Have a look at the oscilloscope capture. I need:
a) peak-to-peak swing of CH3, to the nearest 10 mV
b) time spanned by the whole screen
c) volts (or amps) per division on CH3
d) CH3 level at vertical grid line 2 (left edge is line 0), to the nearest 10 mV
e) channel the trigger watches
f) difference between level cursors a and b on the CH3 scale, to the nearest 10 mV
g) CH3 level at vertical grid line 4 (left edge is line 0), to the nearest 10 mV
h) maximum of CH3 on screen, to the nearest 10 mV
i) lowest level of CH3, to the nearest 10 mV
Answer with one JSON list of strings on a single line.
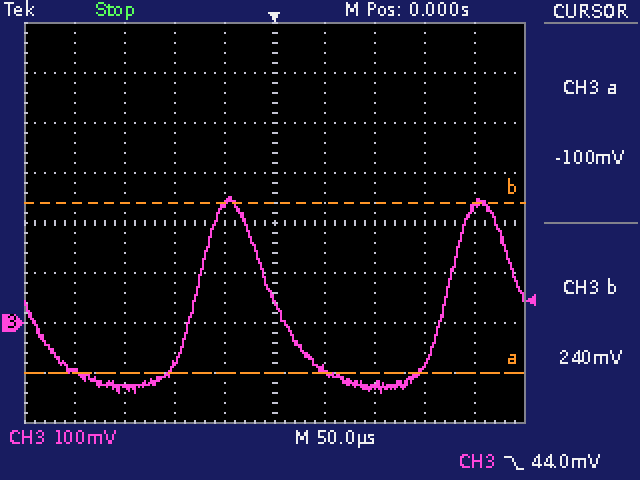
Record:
["390 mV", "500 µs", "100 mV", "-130 mV", "CH3", "340 mV", "240 mV", "250 mV", "-140 mV"]
